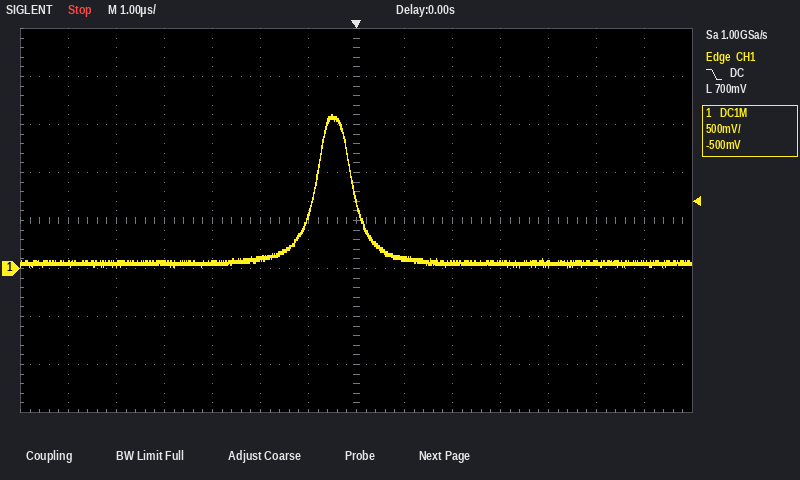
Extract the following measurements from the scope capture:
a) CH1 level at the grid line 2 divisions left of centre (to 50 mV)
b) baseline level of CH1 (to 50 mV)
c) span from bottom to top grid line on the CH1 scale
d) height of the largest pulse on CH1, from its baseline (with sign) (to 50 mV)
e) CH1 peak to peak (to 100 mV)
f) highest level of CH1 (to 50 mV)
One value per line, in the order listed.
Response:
100 mV
50 mV
4 V
+1.55 V
1.60 V
1.60 V
